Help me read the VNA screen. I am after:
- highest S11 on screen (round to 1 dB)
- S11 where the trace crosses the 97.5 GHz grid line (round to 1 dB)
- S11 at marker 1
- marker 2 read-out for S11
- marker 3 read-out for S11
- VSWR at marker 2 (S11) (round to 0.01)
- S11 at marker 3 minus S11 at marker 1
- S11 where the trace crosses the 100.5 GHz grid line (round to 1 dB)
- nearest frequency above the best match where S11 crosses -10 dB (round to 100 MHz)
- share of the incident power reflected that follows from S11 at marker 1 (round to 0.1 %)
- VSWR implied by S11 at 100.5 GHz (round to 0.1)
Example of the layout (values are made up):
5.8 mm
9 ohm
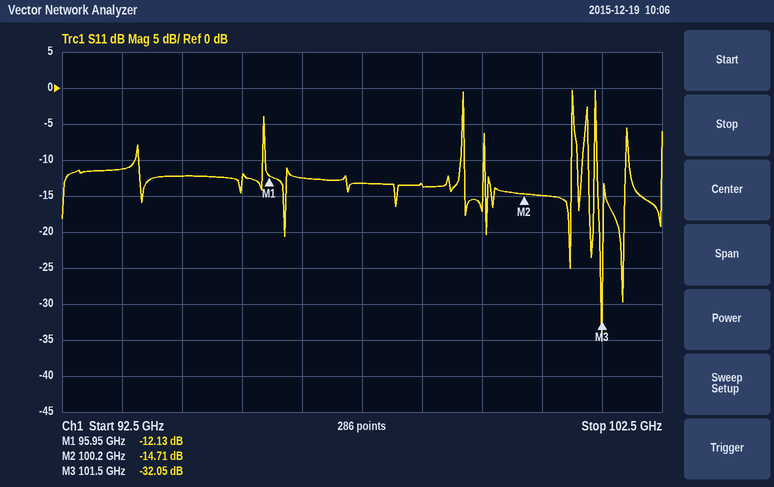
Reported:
0 dB
-13 dB
-12.13 dB
-14.71 dB
-32.05 dB
1.45
-19.92 dB
-15 dB
101.9 GHz
6.1 %
1.4
